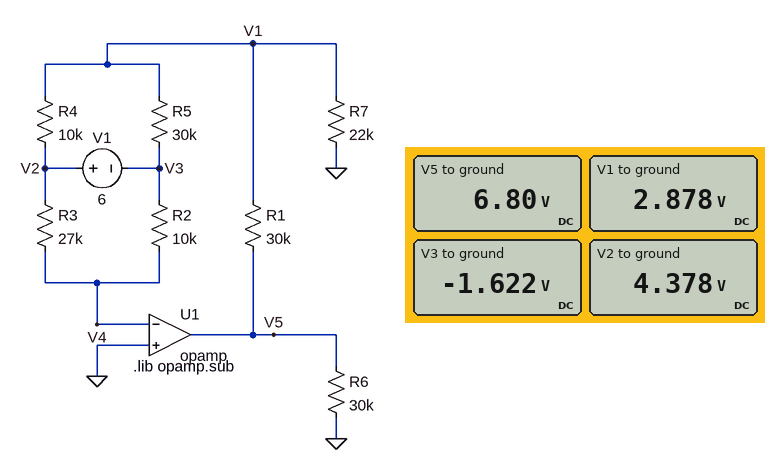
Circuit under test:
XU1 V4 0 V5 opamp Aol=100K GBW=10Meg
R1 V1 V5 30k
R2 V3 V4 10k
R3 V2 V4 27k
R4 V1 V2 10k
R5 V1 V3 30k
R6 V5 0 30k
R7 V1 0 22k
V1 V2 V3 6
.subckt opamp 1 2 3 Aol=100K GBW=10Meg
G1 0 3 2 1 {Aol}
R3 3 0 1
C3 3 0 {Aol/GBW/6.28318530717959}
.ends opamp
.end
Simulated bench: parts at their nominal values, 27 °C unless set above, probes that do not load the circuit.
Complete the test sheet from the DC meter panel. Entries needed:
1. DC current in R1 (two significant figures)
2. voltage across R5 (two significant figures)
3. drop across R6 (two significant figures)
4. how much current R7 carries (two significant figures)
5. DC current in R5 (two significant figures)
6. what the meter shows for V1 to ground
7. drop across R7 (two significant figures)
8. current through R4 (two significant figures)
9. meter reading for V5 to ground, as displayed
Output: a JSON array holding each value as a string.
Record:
["130 µA", "4.5 V", "6.8 V", "130 µA", "150 µA", "2.878 V", "2.9 V", "150 µA", "6.80 V"]
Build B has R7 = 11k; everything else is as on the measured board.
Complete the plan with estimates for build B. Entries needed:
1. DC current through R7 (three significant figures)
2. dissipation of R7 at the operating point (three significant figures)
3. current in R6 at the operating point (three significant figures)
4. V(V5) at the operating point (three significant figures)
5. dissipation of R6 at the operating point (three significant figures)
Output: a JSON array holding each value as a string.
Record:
["262 µA", "753 µW", "358 µA", "10.7 V", "3.84 mW"]
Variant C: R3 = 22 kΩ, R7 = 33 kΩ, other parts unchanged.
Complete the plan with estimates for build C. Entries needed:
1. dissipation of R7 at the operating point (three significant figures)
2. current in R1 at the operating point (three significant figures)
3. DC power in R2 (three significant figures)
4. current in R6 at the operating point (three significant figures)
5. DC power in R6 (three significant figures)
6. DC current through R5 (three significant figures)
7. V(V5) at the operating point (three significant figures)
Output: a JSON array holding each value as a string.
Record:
["209 µW", "79.5 µA", "352 µW", "167 µA", "837 µW", "150 µA", "5.01 V"]
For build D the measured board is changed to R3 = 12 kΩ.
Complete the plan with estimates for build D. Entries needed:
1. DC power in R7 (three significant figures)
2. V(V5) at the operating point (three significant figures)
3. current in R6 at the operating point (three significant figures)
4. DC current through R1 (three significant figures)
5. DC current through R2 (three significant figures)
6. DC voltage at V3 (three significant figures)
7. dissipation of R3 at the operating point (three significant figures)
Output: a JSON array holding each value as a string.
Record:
["143 µW", "4.19 V", "140 µA", "80.6 µA", "273 µA", "-2.73 V", "893 µW"]
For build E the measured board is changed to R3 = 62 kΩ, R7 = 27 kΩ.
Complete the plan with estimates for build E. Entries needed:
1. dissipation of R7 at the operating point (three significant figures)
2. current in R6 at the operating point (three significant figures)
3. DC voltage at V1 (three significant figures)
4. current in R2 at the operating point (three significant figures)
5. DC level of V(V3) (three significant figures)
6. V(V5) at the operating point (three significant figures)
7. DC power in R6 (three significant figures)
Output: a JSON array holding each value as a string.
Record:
["498 µW", "258 µA", "3.67 V", "83.3 µA", "-833 mV", "7.74 V", "2.00 mW"]
